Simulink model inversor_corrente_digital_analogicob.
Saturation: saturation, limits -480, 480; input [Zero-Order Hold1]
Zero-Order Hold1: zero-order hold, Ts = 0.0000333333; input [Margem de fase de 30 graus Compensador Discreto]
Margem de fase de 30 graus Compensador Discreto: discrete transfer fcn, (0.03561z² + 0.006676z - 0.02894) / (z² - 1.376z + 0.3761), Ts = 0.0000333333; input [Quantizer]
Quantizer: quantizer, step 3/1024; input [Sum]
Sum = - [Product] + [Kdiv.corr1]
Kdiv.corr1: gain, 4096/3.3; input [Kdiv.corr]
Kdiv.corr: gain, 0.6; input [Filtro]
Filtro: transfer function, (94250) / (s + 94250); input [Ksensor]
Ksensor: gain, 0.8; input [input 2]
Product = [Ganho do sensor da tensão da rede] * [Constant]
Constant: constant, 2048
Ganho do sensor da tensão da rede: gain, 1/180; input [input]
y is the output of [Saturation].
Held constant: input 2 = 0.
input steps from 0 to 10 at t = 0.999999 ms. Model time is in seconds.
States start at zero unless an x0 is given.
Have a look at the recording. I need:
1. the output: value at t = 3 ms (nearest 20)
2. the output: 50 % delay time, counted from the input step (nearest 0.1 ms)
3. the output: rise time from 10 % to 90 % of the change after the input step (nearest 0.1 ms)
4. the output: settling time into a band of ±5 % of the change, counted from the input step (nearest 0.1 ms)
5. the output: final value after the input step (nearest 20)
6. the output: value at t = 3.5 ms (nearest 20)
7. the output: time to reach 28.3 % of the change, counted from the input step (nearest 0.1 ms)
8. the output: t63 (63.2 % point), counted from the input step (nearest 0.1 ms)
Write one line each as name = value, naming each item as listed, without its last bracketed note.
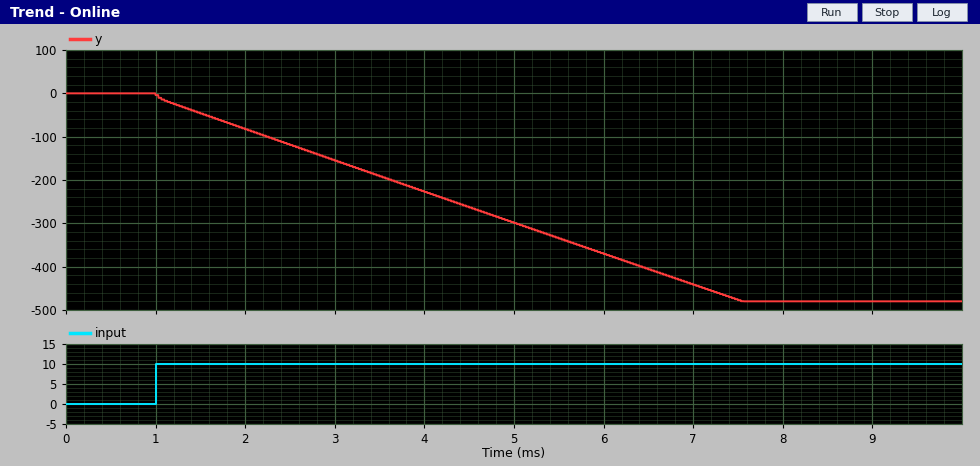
the output: value at t = 3 ms = -160
the output: 50 % delay time, counted from the input step = 3.2 ms
the output: rise time from 10 % to 90 % of the change after the input step = 5.3 ms
the output: settling time into a band of ±5 % of the change, counted from the input step = 6.2 ms
the output: final value after the input step = -480
the output: value at t = 3.5 ms = -200
the output: time to reach 28.3 % of the change, counted from the input step = 1.7 ms
the output: t63 (63.2 % point), counted from the input step = 4.1 ms
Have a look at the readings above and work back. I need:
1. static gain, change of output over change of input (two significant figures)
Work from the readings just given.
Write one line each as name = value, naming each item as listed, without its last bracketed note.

static gain, change of output over change of input = -48
